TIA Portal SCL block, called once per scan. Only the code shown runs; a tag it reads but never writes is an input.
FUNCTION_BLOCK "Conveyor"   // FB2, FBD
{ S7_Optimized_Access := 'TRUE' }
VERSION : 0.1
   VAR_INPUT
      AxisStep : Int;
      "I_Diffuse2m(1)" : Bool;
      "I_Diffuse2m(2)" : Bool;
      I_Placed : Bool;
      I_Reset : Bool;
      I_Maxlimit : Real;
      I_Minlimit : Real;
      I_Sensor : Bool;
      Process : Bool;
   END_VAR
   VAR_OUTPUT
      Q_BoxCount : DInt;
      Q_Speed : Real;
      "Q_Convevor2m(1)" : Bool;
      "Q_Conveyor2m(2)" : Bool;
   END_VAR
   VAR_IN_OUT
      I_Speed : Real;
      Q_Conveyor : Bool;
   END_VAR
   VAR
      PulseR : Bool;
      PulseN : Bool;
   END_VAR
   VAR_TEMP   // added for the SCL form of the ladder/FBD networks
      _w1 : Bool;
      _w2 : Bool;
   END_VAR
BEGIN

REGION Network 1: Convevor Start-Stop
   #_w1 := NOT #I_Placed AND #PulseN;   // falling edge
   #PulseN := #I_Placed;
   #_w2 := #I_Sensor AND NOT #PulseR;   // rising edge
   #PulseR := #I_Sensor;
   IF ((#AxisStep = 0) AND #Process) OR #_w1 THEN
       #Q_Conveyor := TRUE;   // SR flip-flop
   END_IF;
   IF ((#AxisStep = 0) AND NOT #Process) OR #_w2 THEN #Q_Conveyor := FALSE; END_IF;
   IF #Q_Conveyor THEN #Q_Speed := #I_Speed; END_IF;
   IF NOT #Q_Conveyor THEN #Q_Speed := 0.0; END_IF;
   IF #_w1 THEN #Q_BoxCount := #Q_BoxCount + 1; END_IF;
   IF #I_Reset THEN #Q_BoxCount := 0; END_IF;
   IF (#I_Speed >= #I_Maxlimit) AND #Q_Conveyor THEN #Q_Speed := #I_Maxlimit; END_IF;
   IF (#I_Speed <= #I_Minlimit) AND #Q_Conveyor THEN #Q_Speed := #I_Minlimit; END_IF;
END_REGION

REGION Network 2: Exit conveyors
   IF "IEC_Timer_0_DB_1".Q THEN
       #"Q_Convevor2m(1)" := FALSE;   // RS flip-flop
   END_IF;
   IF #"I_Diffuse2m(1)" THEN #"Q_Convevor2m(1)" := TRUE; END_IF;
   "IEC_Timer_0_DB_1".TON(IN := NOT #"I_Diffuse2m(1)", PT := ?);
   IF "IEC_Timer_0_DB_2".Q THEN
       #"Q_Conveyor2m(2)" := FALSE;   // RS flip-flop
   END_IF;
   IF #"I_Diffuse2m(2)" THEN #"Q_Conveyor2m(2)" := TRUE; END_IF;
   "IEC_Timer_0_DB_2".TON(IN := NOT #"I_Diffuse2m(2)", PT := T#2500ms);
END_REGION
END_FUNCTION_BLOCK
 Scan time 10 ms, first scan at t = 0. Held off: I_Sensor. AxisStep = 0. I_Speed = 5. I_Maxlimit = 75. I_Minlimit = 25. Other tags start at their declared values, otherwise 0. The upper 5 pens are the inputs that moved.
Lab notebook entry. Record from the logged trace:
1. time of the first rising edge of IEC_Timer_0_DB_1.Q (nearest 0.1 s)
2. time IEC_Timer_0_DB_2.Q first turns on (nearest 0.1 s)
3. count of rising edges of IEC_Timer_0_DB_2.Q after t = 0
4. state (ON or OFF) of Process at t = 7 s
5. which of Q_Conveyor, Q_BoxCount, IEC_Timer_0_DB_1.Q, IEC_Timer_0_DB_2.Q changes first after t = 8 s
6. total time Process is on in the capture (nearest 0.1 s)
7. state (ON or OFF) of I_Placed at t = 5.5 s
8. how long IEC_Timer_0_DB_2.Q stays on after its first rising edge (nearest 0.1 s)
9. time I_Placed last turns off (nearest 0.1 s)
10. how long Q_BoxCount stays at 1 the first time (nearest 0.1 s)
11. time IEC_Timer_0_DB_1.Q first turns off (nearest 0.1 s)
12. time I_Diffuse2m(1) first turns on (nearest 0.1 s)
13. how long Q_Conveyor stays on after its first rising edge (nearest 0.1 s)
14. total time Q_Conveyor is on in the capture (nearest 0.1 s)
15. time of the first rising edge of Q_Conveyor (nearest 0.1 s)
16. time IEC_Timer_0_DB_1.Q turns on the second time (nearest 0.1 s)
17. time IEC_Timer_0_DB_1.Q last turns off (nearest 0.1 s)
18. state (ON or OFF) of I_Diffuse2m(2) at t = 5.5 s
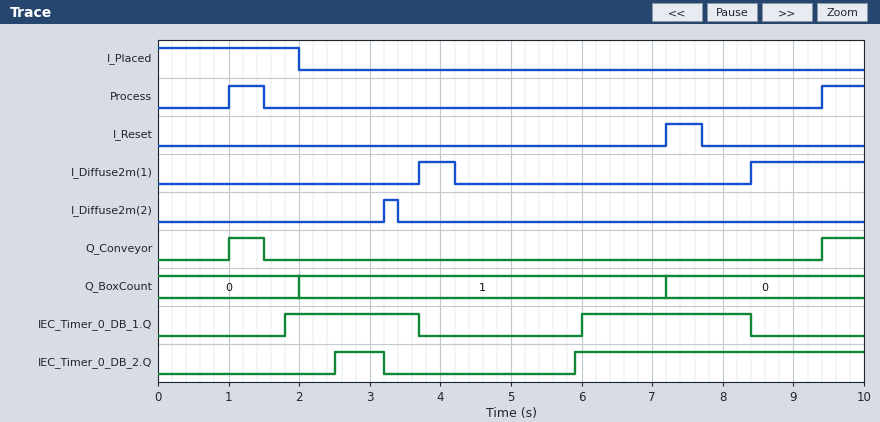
1.8 s
2.5 s
2
OFF
IEC_Timer_0_DB_1.Q
1.1 s
OFF
0.7 s
2.0 s
5.2 s
3.7 s
3.7 s
0.5 s
1.1 s
1.0 s
6.0 s
8.4 s
OFF
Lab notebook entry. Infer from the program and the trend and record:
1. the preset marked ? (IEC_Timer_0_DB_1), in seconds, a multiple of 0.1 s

1.8 s
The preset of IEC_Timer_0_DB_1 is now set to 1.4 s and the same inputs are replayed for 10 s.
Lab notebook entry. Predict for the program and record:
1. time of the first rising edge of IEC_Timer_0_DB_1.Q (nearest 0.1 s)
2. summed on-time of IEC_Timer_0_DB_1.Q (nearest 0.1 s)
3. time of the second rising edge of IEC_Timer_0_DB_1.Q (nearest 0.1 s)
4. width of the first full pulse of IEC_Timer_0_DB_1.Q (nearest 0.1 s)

1.4 s
5.1 s
5.6 s
2.3 s
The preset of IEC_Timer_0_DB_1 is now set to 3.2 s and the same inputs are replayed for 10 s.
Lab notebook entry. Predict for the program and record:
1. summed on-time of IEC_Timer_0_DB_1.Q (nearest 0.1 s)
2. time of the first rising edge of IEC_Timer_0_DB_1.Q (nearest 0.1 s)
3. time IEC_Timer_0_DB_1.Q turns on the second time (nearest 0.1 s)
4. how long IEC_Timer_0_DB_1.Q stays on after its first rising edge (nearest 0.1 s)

1.5 s
3.2 s
7.4 s
0.5 s
